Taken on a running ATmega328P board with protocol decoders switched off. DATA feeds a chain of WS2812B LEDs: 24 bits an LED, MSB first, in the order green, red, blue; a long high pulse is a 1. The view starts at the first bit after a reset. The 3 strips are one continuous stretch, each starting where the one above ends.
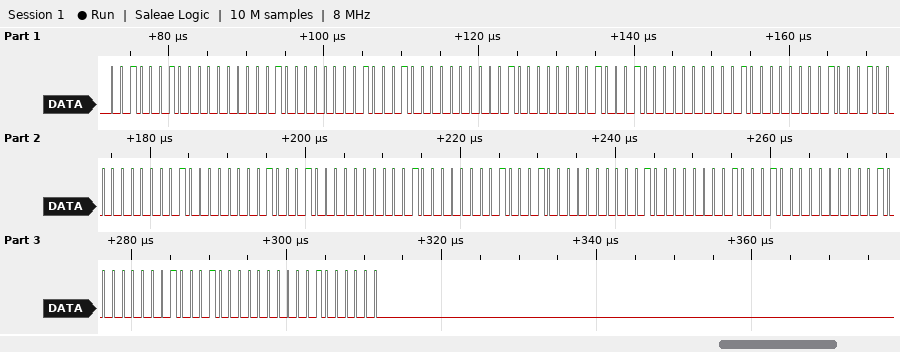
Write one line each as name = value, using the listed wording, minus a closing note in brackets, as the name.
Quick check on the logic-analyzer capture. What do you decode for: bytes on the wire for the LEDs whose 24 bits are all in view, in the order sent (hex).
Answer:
bytes on the wire for the LEDs whose 24 bits are all in view, in the order sent = 22 00 40 22 00 40 22 00 40 22 00 40 22 00 40 22 00 40 22 00 40 22 00 40
